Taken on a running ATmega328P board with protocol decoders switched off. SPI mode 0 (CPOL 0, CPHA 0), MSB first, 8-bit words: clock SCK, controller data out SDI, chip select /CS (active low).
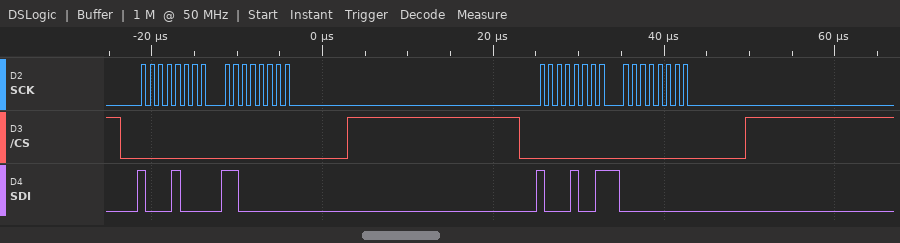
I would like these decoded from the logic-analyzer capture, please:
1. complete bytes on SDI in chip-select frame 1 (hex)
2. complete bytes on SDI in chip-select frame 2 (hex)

88 C0
89 00
